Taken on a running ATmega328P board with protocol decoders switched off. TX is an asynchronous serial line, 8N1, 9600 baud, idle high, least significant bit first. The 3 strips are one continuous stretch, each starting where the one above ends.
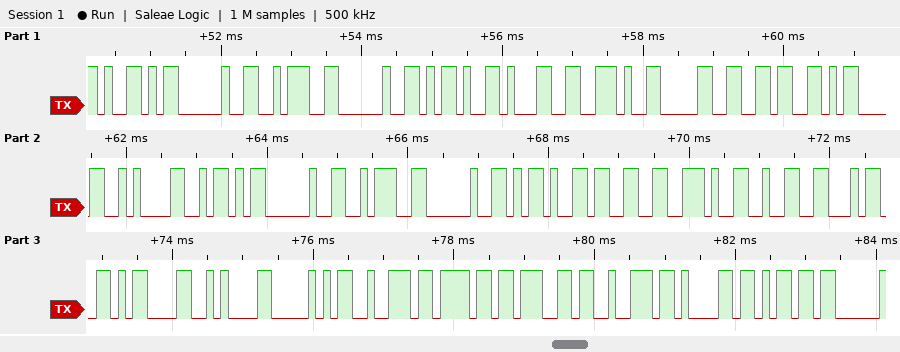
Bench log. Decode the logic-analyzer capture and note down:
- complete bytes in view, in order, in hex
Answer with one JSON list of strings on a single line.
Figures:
["0x59 0x20 0x3A 0x20 0x2D 0x31 0x2E 0x30 0x36 0x0D 0x0A 0x5A 0x20 0x3A 0x20 0x2D 0x33 0x2E 0x32 0x34 0x0D 0x0A 0x50 0x72 0x6F 0x67 0x72 0x61 0x6D"]
